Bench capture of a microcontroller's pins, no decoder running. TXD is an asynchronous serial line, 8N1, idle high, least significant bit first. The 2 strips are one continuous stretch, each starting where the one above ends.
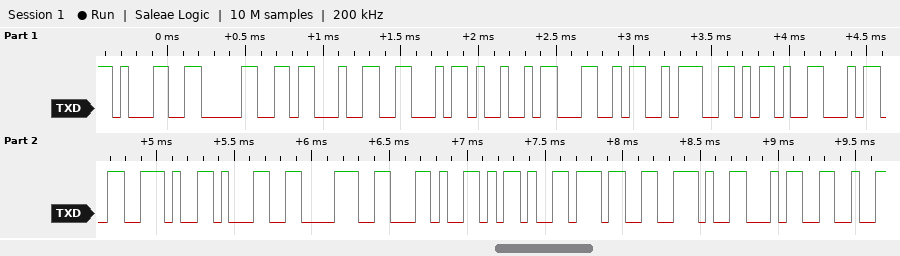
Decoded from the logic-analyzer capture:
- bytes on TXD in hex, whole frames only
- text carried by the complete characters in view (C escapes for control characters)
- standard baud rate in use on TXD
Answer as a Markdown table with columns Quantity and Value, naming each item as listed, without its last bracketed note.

| Quantity | Value |
|---|---|
| bytes on TXD in hex, whole frames only | 0x31 0x30 0x23 0x46 0x49 0x4C 0x3A 0x2D 0x34 0x2E 0x31 0x38 0x2C 0x2D 0x37 0x2E 0x34 |
| text carried by the complete characters in view | "10#FIL:-4.18,-7.4" |
| standard baud rate in use on TXD | 19200 baud |
